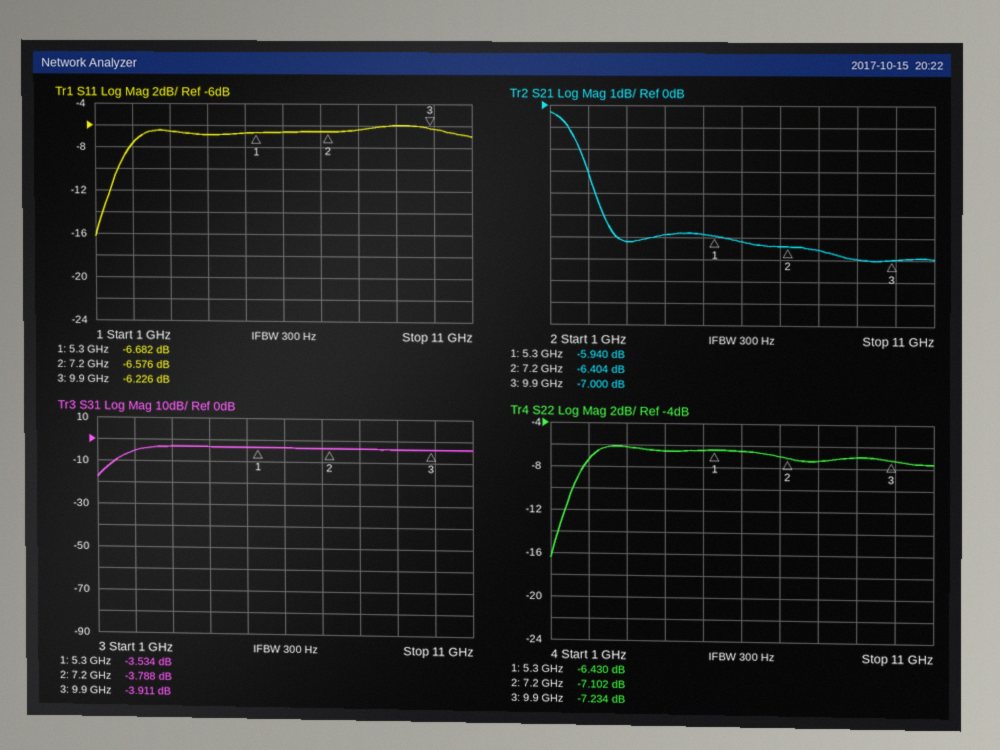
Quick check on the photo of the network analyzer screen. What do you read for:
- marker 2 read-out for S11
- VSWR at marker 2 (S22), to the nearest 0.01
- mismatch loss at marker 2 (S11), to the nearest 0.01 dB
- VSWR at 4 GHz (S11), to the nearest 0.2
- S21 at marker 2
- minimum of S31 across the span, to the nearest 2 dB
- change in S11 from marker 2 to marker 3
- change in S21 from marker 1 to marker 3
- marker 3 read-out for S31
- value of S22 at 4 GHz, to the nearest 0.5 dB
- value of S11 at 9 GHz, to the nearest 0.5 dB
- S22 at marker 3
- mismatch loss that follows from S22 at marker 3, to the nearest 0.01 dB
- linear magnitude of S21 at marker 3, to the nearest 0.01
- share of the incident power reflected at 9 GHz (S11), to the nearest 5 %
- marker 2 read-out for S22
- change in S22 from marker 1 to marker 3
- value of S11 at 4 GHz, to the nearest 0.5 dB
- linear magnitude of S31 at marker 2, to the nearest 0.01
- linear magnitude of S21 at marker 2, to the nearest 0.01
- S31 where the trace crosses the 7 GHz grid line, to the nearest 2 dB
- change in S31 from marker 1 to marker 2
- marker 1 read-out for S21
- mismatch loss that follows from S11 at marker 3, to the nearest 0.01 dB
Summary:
-6.576 dB
2.58
1.08 dB
2.6
-6.404 dB
-18 dB
0.350 dB
-1.060 dB
-3.911 dB
-6.5 dB
-6.0 dB
-7.234 dB
0.91 dB
0.45
25 %
-7.102 dB
-0.804 dB
-7.0 dB
0.65
0.48
-4 dB
-0.254 dB
-5.940 dB
1.18 dB
